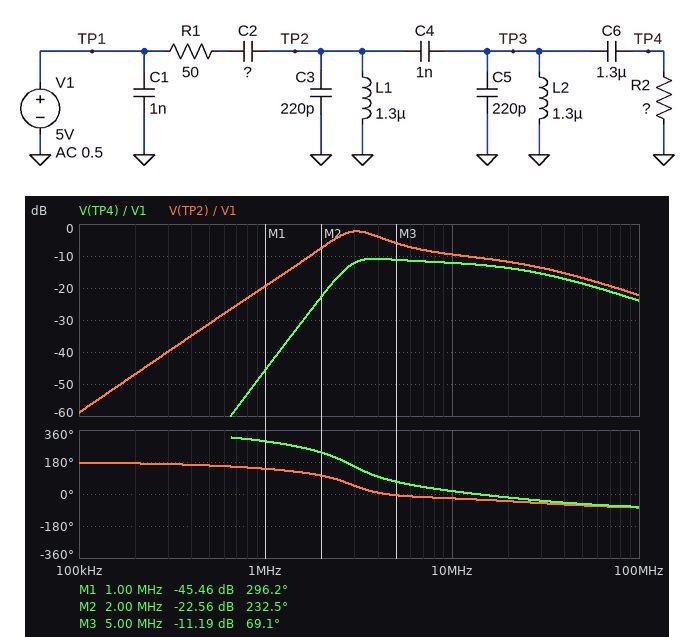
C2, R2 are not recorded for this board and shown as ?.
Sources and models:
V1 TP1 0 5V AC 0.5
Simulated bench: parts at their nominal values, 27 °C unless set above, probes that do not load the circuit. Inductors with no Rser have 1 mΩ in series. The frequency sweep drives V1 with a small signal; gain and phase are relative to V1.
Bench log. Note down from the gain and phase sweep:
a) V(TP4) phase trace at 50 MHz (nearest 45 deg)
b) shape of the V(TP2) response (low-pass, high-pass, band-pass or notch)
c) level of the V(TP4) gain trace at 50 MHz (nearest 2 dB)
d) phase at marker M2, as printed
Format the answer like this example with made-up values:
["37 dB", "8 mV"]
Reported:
["-45 deg", "band-pass", "-18 dB", "232.5 deg"]
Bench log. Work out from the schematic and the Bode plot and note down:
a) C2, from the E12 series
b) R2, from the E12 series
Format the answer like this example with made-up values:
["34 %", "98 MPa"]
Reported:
["2.2 nF", "18 Ω"]
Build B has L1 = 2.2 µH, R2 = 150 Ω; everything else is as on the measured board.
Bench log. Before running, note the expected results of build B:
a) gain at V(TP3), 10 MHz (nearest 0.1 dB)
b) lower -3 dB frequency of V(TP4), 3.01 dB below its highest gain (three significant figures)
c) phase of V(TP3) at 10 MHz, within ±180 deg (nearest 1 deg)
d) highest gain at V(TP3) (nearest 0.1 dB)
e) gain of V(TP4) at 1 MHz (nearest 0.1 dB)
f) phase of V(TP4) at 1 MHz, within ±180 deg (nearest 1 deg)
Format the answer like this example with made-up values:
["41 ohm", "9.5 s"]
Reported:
["-3.4 dB", "3.45 MHz", "-10 deg", "-1.9 dB", "-39.0 dB", "-45 deg"]
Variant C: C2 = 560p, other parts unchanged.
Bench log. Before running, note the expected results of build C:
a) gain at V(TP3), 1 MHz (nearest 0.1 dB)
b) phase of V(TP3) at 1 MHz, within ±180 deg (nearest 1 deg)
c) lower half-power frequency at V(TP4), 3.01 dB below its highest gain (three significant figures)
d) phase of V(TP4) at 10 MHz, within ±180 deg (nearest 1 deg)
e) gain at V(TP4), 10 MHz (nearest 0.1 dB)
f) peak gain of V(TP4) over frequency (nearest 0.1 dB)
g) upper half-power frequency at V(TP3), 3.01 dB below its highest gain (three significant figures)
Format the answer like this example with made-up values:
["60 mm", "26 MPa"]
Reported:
["-56.2 dB", "-36 deg", "2.91 MHz", "31 deg", "-13.3 dB", "-10.6 dB", "15.0 MHz"]
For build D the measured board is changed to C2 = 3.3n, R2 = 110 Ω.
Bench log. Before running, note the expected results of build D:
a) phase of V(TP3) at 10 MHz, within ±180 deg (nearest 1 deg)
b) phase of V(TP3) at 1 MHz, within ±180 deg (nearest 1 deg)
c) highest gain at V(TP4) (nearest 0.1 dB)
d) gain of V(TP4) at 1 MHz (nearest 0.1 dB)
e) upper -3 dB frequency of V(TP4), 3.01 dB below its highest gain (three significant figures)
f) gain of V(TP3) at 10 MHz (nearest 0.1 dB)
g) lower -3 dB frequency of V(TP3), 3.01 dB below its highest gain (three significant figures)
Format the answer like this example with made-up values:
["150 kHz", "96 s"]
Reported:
["1 deg", "-56 deg", "-3.1 dB", "-42.5 dB", "14.4 MHz", "-3.6 dB", "2.65 MHz"]
